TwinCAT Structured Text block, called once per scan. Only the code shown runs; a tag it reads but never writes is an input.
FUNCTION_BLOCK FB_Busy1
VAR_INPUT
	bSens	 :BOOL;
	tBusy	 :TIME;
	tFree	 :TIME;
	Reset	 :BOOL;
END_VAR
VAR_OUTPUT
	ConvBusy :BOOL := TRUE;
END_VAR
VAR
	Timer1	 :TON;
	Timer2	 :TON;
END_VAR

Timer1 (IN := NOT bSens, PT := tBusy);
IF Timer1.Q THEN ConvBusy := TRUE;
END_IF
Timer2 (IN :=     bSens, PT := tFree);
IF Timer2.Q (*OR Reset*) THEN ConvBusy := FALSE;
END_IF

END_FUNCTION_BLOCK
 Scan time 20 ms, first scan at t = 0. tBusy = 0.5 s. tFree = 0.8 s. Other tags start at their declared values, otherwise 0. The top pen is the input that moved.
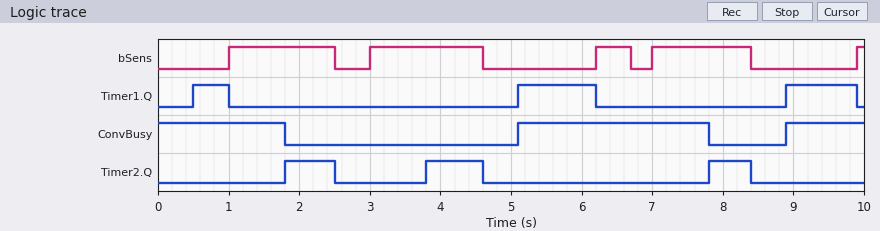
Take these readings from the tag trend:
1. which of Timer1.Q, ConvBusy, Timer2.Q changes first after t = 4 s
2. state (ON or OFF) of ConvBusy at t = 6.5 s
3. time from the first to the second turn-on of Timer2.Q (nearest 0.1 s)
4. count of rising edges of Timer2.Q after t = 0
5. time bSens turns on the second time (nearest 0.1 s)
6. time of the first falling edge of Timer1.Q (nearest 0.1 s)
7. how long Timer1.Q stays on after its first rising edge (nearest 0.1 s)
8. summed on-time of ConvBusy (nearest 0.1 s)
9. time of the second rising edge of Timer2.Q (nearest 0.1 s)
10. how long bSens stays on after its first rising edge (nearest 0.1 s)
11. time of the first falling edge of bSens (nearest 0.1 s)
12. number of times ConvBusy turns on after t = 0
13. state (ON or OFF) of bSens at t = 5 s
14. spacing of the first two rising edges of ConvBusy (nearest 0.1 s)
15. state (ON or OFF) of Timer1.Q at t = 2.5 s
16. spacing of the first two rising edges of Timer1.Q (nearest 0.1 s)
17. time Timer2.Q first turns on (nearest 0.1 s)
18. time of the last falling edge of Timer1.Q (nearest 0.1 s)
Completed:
Timer2.Q
ON
2.0 s
3
3.0 s
1.0 s
0.5 s
5.6 s
3.8 s
1.5 s
2.5 s
2
OFF
3.8 s
OFF
4.6 s
1.8 s
9.9 s
